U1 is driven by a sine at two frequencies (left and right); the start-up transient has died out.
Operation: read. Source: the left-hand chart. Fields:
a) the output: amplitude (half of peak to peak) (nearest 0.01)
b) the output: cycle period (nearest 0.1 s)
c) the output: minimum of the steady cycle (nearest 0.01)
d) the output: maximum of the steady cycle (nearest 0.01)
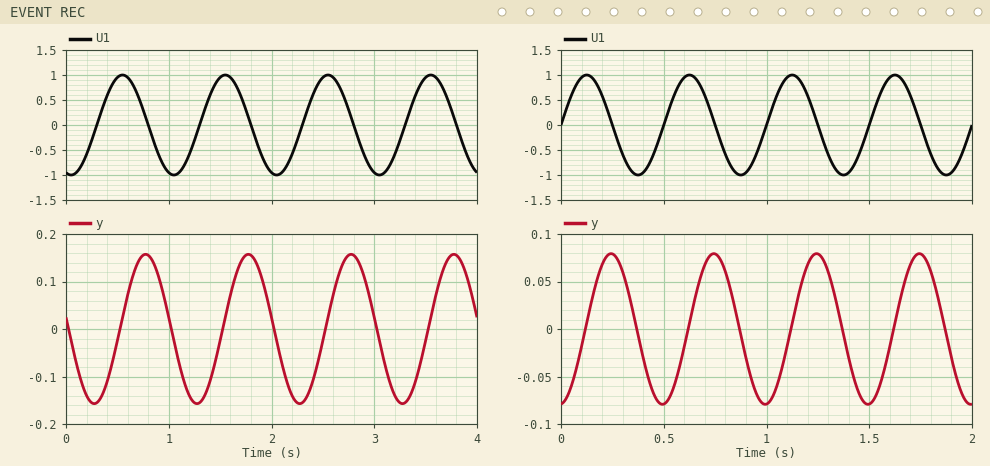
0.16
1.0 s
-0.16
0.16
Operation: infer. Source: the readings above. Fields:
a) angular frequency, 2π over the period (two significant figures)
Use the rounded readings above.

6.3 rad/s
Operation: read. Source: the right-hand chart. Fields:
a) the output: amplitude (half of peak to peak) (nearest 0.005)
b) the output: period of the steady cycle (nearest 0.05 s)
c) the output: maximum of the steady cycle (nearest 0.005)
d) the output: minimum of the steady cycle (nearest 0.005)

0.080
0.50 s
0.080
-0.080
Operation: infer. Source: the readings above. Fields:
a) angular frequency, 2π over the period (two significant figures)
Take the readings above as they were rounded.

13 rad/s
